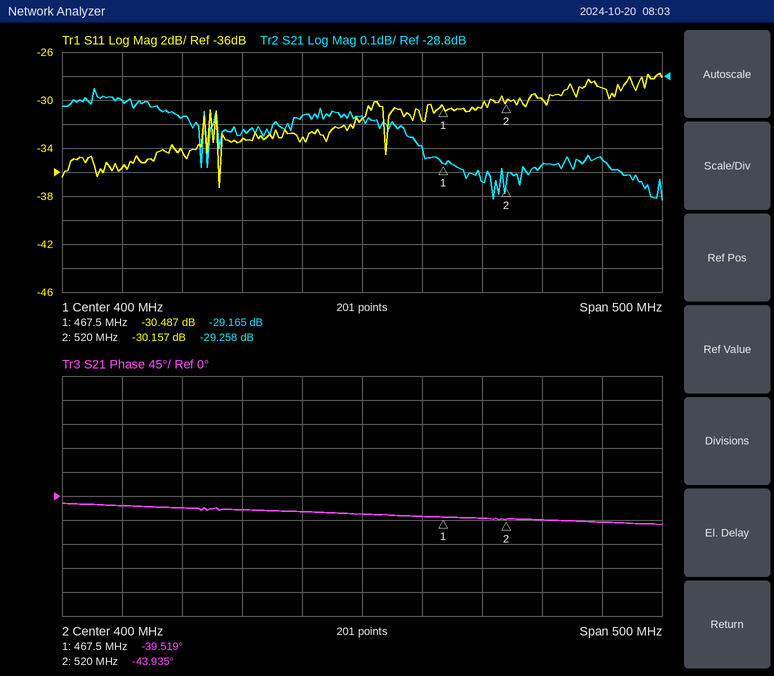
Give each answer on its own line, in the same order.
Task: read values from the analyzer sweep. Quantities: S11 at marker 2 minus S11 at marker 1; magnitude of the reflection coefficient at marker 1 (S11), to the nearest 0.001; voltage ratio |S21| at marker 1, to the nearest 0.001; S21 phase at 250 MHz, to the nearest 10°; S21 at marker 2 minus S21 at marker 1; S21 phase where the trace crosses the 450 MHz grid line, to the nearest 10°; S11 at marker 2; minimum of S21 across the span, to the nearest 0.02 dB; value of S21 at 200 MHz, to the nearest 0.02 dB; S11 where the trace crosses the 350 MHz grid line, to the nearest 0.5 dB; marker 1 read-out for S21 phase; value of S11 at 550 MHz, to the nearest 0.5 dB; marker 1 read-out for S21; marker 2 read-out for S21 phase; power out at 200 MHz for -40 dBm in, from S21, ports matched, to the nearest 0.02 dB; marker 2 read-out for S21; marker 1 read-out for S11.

0.330 dB
0.030
0.035
-20°
-0.093 dB
-40°
-30.157 dB
-29.32 dB
-28.90 dB
-33.0 dB
-39.519°
-30.0 dB
-29.165 dB
-43.935°
-68.90 dBm
-29.258 dB
-30.487 dB
